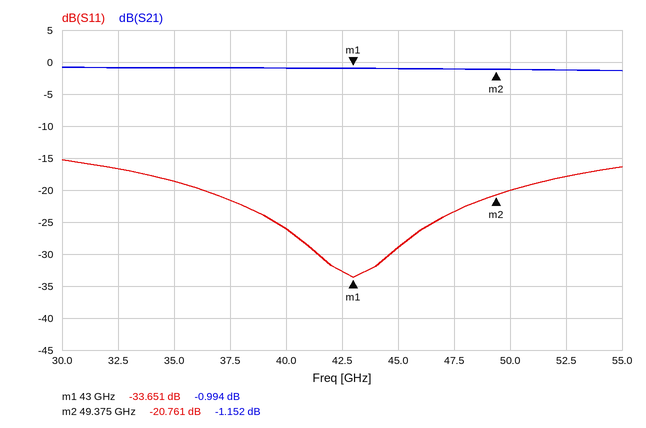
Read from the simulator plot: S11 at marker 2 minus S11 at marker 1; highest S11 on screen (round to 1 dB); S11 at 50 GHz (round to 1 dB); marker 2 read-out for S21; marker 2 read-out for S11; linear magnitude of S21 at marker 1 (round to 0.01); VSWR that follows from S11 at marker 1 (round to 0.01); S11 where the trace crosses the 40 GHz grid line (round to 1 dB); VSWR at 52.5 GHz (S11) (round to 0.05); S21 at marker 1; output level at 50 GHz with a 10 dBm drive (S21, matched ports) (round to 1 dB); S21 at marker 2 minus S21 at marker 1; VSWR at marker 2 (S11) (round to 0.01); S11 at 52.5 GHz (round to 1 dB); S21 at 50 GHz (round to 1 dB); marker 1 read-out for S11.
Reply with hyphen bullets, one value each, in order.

- 12.890 dB
- -15 dB
- -20 dB
- -1.152 dB
- -20.761 dB
- 0.89
- 1.04
- -26 dB
- 1.30
- -0.994 dB
- 9 dBm
- -0.158 dB
- 1.20
- -18 dB
- -1 dB
- -33.651 dB
